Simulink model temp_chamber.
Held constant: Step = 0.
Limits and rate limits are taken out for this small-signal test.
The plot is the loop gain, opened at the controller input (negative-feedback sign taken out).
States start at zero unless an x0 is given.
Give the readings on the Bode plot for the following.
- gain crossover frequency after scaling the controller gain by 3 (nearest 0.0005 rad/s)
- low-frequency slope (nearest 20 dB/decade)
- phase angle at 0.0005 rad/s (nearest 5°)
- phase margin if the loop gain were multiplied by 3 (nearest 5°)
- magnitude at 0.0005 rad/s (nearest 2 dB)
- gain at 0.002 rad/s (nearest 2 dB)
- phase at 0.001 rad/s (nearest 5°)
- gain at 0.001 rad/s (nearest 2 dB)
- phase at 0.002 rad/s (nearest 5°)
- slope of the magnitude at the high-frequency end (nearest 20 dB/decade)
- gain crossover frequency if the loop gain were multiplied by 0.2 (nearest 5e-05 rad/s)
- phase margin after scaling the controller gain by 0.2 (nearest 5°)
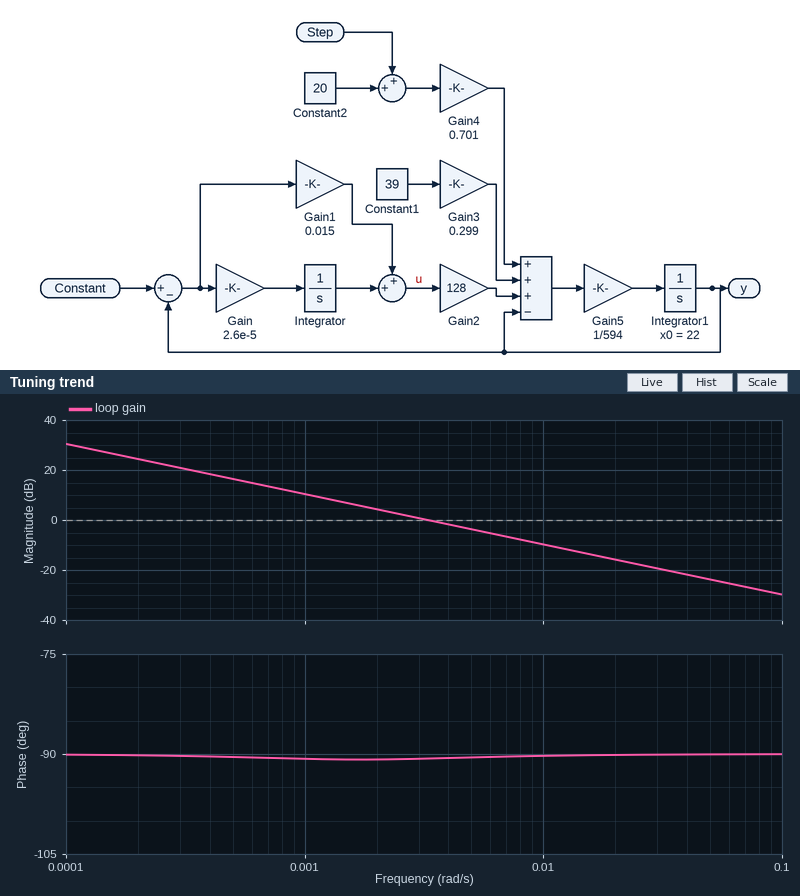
0.0095 rad/s
-20 dB/decade
-90°
90°
16 dB
4 dB
-90°
10 dB
-90°
-20 dB/decade
0.00065 rad/s
90°
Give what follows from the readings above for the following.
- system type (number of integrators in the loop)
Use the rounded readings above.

1
